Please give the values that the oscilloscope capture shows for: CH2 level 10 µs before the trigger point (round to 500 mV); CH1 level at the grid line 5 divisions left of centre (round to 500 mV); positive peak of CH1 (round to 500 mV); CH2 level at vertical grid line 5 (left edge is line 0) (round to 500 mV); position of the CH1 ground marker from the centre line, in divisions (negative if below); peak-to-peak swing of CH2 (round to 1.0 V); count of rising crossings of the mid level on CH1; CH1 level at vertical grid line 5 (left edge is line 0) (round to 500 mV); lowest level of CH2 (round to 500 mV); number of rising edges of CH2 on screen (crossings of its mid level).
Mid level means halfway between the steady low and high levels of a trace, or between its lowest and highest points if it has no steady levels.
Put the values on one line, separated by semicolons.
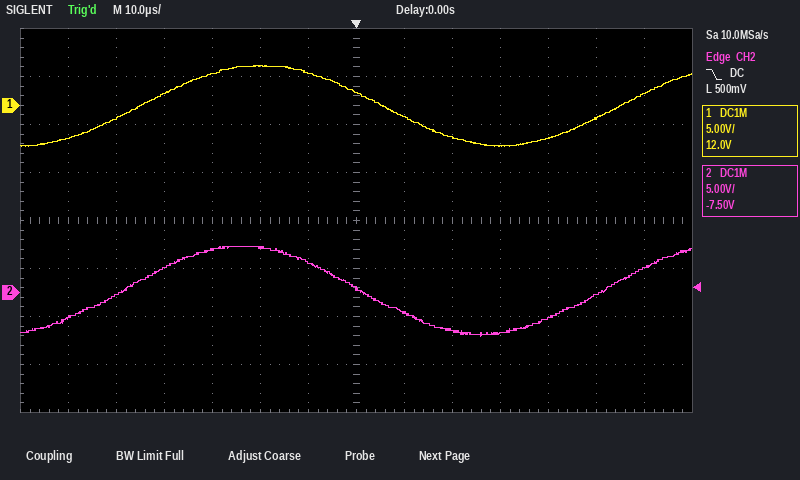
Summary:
3.0 V; -1.5 V; 4.0 V; 4.5 V; +2.4 div; 9.0 V; 2; 4.0 V; -4.5 V; 2
